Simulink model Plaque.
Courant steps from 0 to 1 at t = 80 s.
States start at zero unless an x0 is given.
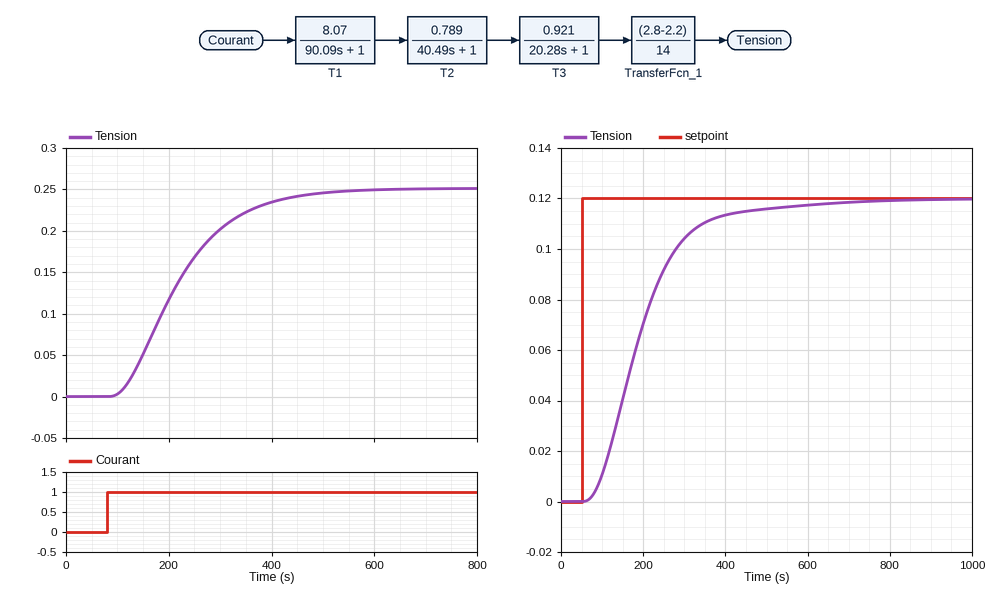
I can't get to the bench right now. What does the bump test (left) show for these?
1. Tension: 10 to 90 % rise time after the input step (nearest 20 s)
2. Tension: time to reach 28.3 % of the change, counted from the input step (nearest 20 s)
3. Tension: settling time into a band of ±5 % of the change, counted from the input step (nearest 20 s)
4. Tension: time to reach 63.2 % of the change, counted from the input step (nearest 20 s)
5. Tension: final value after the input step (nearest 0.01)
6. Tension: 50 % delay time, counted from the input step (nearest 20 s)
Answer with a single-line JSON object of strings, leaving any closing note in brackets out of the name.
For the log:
{"Tension: 10 to 90 % rise time after the input step": "240 s", "Tension: time to reach 28.3 % of the change, counted from the input step": "80 s", "Tension: settling time into a band of ±5 % of the change, counted from the input step": "340 s", "Tension: time to reach 63.2 % of the change, counted from the input step": "160 s", "Tension: final value after the input step": "0.25", "Tension: 50 % delay time, counted from the input step": "120 s"}
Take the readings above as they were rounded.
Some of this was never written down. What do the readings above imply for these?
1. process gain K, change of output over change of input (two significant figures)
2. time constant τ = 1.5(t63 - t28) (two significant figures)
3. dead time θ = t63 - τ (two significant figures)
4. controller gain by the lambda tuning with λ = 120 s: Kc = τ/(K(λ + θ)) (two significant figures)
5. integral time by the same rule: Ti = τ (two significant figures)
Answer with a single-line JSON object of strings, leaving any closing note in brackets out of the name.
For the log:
{"process gain K, change of output over change of input": "0.25", "time constant τ = 1.5(t63 - t28)": "120 s", "dead time θ = t63 - τ": "40 s", "controller gain by the lambda tuning with λ = 120 s: Kc = τ/(K(λ + θ))": "3.0", "integral time by the same rule: Ti = τ": "120 s"}
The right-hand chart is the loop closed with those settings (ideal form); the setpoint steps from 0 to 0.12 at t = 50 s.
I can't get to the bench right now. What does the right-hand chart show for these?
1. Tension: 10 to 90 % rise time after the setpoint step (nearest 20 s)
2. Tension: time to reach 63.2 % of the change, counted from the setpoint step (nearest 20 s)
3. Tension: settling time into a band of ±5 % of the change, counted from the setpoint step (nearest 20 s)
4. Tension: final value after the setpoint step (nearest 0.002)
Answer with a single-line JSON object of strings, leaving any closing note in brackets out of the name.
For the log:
{"Tension: 10 to 90 % rise time after the setpoint step": "220 s", "Tension: time to reach 63.2 % of the change, counted from the setpoint step": "160 s", "Tension: settling time into a band of ±5 % of the change, counted from the setpoint step": "360 s", "Tension: final value after the setpoint step": "0.120"}
